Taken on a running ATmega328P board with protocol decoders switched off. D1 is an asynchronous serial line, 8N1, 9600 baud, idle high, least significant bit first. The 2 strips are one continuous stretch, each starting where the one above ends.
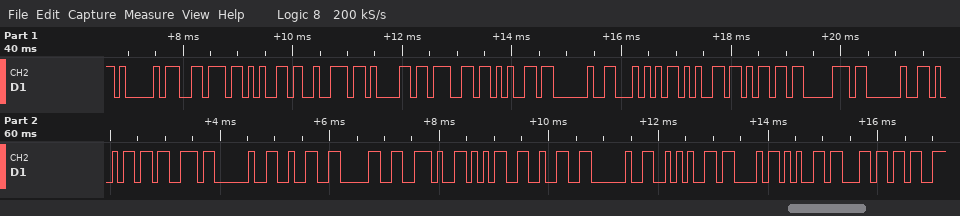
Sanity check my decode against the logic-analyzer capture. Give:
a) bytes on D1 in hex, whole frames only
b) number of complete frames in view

41 76 65 72 61 67 65 20 54 65 6D 70 20 69 73 20 32 30 2E 35 32 20 2A 43 65 6C
26
